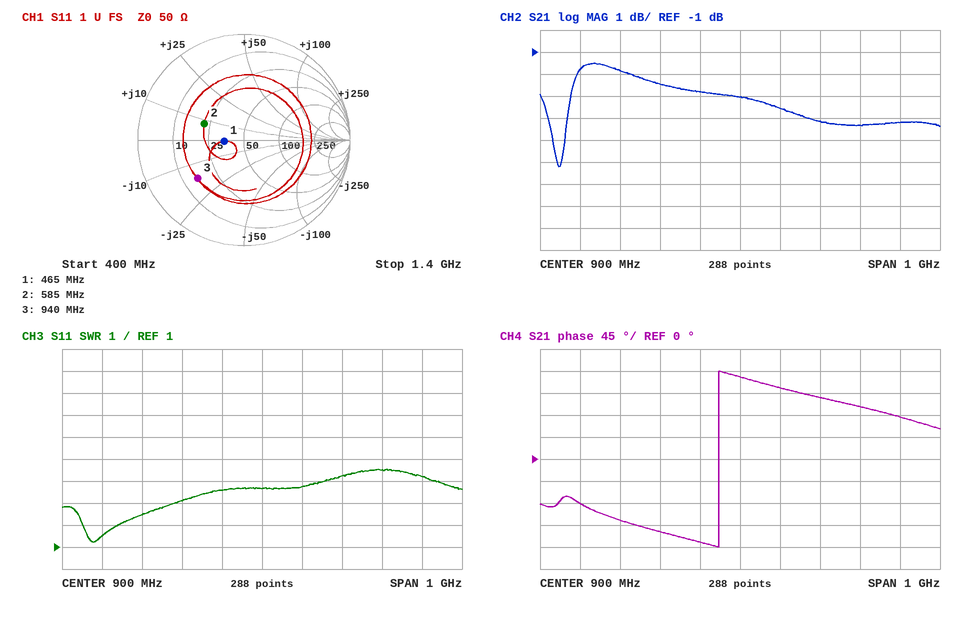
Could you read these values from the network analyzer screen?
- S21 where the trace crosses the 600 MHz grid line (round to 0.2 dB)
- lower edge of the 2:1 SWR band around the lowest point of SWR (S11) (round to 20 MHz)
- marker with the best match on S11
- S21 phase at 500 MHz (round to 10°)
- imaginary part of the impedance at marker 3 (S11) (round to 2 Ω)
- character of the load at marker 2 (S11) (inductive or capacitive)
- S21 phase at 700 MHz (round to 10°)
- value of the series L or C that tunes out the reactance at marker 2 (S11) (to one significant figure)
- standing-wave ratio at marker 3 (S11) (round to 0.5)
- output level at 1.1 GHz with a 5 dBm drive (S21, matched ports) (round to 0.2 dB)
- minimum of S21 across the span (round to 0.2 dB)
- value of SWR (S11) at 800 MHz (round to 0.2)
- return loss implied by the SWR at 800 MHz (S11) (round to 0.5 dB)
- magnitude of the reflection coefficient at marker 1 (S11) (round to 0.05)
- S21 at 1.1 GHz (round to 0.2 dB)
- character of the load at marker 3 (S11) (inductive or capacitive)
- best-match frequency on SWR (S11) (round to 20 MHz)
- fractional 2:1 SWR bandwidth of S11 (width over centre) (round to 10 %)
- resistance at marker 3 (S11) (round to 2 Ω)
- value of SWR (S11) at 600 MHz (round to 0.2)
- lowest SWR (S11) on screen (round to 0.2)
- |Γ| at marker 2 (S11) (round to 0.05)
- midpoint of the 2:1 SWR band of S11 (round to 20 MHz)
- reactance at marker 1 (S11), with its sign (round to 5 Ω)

-1.8 dB
460 MHz
marker 1
-90°
-16 Ω
inductive
-150°
30 pF
3.5
0.8 dBm
-6.2 dB
3.6
5.0 dB
0.20
-4.2 dB
capacitive
480 MHz
20 %
16 Ω
2.4
1.2
0.40
500 MHz
0 Ω
